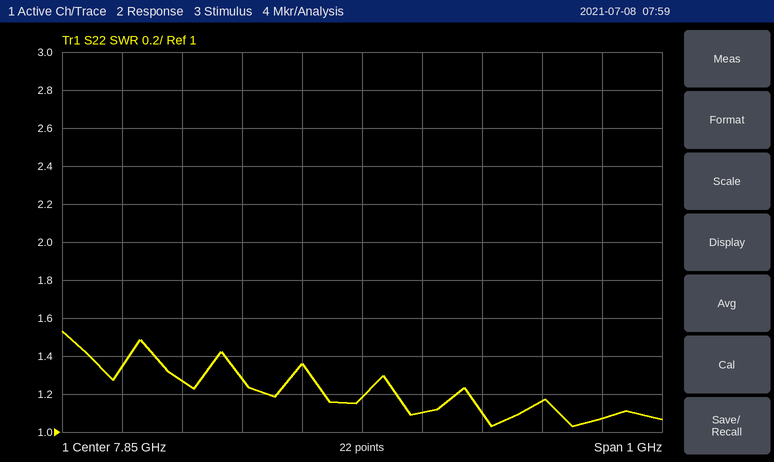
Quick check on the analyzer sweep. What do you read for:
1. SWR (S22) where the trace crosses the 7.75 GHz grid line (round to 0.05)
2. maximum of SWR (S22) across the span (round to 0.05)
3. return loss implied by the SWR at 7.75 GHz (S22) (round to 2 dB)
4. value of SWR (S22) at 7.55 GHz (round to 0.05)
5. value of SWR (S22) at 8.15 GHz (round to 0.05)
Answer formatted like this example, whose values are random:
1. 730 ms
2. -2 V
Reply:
1. 1.35
2. 1.55
3. 16 dB
4. 1.25
5. 1.15
